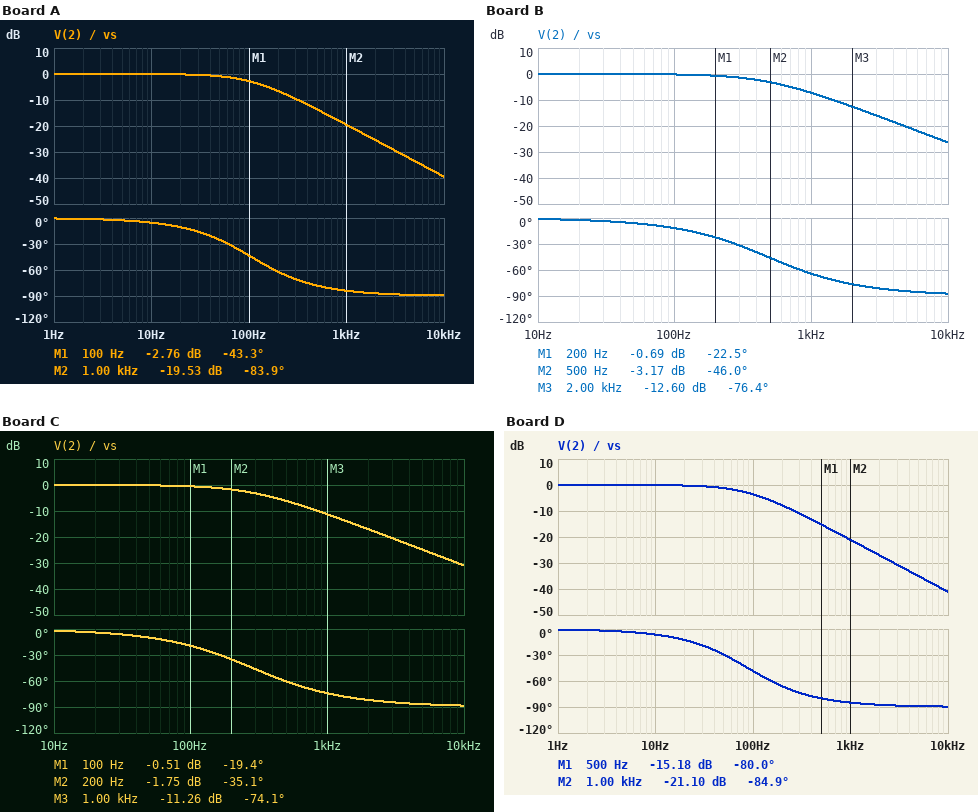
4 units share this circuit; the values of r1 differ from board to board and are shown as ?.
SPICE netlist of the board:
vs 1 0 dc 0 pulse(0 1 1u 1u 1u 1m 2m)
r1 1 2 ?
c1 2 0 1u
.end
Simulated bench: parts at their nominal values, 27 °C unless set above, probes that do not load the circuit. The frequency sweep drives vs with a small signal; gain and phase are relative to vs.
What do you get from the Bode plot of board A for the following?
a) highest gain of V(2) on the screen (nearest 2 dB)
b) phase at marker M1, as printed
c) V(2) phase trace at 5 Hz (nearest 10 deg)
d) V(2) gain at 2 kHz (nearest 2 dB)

0 dB
-43.3 deg
0 deg
-26 dB
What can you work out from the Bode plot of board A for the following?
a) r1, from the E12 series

1.5 kΩ
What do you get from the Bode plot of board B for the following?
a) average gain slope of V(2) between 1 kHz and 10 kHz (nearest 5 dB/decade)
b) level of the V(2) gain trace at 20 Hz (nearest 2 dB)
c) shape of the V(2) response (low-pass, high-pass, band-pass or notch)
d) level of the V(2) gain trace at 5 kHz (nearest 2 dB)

-20 dB/decade
0 dB
low-pass
-20 dB
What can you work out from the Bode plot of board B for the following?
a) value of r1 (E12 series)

330 Ω
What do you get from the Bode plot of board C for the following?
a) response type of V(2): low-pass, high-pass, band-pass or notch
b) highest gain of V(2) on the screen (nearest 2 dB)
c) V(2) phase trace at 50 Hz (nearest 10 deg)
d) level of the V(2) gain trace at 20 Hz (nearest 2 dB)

low-pass
0 dB
-10 deg
0 dB
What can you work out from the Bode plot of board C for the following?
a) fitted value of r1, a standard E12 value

560 Ω
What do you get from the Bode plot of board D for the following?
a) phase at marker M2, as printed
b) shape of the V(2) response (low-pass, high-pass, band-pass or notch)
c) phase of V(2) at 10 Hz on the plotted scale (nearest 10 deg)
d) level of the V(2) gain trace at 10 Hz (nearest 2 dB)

-84.9 deg
low-pass
-10 deg
0 dB
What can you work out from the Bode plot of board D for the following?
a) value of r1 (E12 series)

1.8 kΩ
